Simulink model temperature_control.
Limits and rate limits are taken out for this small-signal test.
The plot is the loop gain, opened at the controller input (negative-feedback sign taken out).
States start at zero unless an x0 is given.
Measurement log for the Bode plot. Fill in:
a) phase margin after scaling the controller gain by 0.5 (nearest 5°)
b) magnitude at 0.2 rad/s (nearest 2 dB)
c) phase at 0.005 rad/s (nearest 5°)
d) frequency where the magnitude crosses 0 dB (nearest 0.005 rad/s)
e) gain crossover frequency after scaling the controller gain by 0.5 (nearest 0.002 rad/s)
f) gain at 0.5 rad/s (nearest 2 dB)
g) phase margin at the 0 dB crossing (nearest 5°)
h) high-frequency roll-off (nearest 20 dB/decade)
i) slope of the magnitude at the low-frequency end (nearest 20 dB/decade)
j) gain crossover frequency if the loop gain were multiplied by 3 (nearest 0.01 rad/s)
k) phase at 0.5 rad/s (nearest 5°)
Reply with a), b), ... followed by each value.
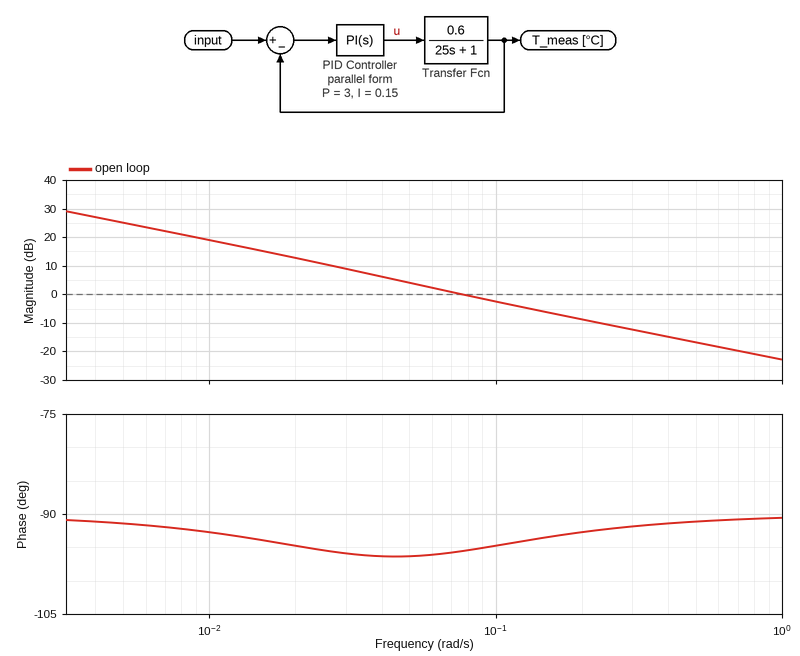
a) 85°
b) -8 dB
c) -90°
d) 0.075 rad/s
e) 0.040 rad/s
f) -16 dB
g) 85°
h) -20 dB/decade
i) -20 dB/decade
j) 0.22 rad/s
k) -90°
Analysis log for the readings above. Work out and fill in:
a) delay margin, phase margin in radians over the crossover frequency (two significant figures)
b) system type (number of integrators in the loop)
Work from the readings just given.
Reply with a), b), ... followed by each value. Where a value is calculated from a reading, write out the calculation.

a) 85 × π / 180 / 0.075 = 20 s
b) 1
